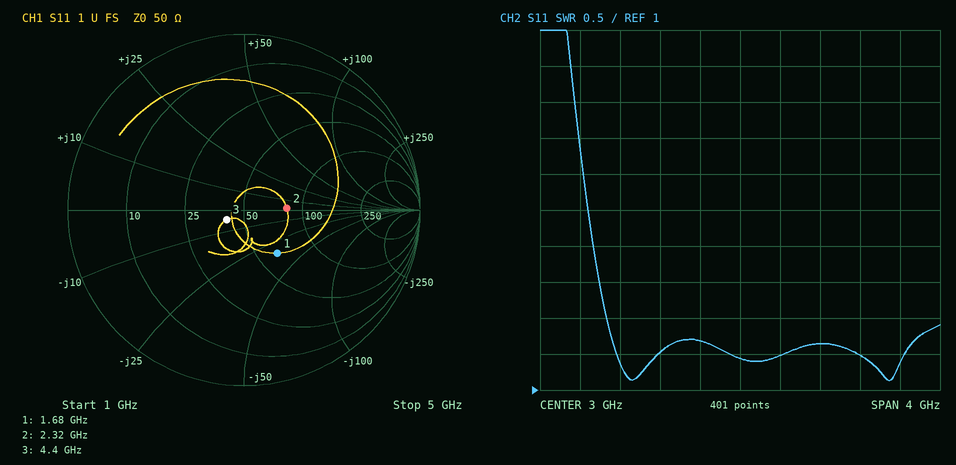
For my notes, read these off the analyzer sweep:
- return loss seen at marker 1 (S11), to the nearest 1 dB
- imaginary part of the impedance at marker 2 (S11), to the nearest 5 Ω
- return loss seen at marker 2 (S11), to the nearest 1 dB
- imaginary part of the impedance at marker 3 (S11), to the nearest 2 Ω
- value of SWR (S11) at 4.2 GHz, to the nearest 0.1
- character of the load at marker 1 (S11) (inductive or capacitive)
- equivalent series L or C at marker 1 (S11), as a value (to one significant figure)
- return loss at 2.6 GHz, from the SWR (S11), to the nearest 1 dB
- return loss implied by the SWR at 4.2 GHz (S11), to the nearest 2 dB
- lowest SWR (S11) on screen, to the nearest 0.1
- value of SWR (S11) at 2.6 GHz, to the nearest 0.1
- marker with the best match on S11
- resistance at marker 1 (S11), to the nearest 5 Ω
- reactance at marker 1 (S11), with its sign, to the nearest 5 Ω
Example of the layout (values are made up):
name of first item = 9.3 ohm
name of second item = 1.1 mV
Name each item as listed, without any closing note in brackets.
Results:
return loss seen at marker 1 (S11), to the nearest 1 dB = 10 dB
imaginary part of the impedance at marker 2 (S11), to the nearest 5 Ω = 0 Ω
return loss seen at marker 2 (S11), to the nearest 1 dB = 12 dB
imaginary part of the impedance at marker 3 (S11), to the nearest 2 Ω = -4 Ω
value of SWR (S11) at 4.2 GHz, to the nearest 0.1 = 1.5
character of the load at marker 1 (S11) = capacitive
equivalent series L or C at marker 1 (S11), as a value = 3 pF
return loss at 2.6 GHz, from the SWR (S11), to the nearest 1 dB = 12 dB
return loss implied by the SWR at 4.2 GHz (S11), to the nearest 2 dB = 14 dB
lowest SWR (S11) on screen, to the nearest 0.1 = 1.1
value of SWR (S11) at 2.6 GHz, to the nearest 0.1 = 1.7
marker with the best match on S11 = marker 3
resistance at marker 1 (S11), to the nearest 5 Ω = 65 Ω
reactance at marker 1 (S11), with its sign, to the nearest 5 Ω = -35 Ω
